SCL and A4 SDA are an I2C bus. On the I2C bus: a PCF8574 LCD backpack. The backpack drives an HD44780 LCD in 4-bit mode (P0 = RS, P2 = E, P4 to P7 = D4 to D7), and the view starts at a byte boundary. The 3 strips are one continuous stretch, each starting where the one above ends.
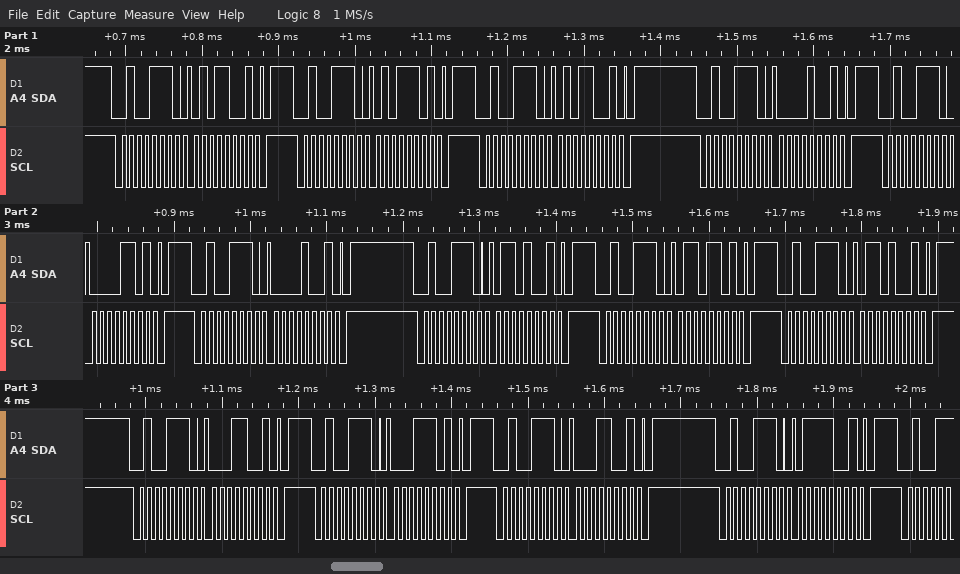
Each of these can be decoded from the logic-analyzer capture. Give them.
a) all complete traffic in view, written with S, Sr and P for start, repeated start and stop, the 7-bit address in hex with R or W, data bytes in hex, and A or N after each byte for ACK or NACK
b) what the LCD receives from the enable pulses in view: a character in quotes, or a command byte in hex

S 27W A 59 A P S 27W A 5D A P S 27W A 59 A P S 27W A 09 A P S 27W A 0D A P S 27W A 09 A P S 27W A 69 A P S 27W A 6D A P S 27W A 69 A P S 27W A 19 A P S 27W A 1D A P S 27W A 19 A P S 27W A 79 A P
'P' 'a'
